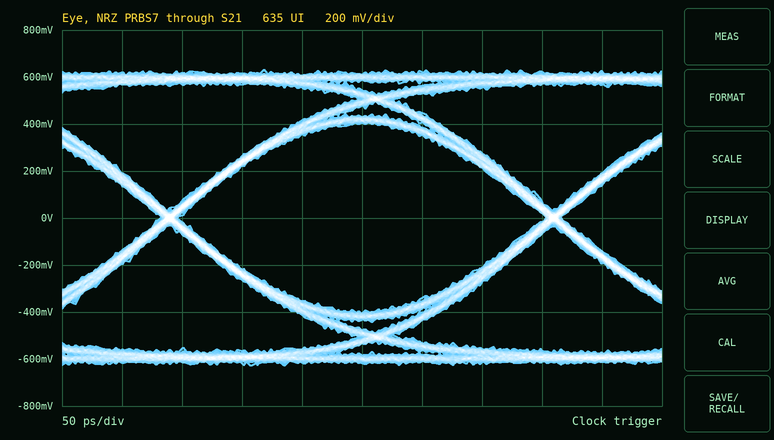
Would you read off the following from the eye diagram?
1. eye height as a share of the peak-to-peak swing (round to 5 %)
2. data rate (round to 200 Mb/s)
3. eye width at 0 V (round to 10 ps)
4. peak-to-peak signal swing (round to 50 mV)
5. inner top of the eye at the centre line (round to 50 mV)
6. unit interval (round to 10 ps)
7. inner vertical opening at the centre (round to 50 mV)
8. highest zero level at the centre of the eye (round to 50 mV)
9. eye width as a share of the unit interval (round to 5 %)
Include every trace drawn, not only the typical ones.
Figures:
65 %
3.2 Gb/s
310 ps
1.25 V
400 mV
320 ps
800 mV
-400 mV
95 %
